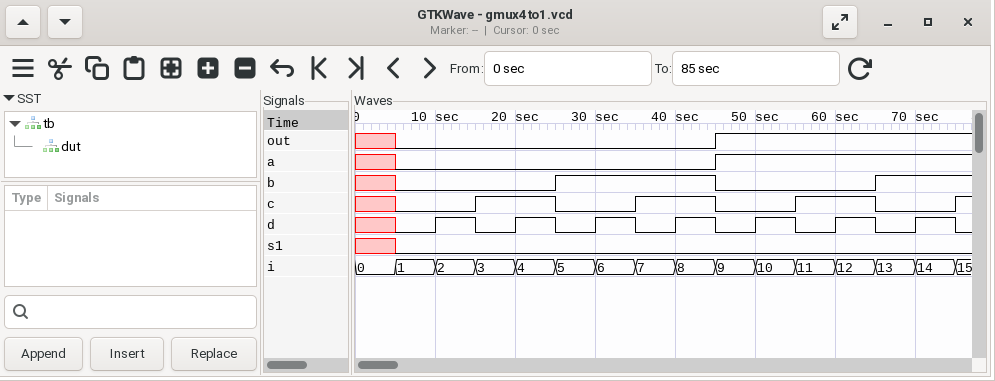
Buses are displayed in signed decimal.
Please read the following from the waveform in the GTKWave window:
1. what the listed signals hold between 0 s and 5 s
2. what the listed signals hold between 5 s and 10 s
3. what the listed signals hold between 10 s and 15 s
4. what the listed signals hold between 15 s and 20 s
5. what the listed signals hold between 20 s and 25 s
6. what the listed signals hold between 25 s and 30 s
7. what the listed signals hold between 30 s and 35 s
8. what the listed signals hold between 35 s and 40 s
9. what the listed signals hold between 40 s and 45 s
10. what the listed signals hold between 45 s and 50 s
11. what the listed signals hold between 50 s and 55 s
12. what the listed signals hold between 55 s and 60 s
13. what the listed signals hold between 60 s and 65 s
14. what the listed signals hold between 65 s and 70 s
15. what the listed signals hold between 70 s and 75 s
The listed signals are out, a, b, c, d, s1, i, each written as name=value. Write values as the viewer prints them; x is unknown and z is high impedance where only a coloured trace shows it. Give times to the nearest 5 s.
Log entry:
out=x, a=x, b=x, c=x, d=x, s1=x, i=0
out=0, a=0, b=0, c=0, d=0, s1=0, i=1
out=0, a=0, b=0, c=0, d=1, s1=0, i=2
out=0, a=0, b=0, c=1, d=0, s1=0, i=3
out=0, a=0, b=0, c=1, d=1, s1=0, i=4
out=0, a=0, b=1, c=0, d=0, s1=0, i=5
out=0, a=0, b=1, c=0, d=1, s1=0, i=6
out=0, a=0, b=1, c=1, d=0, s1=0, i=7
out=0, a=0, b=1, c=1, d=1, s1=0, i=8
out=1, a=1, b=0, c=0, d=0, s1=0, i=9
out=1, a=1, b=0, c=0, d=1, s1=0, i=10
out=1, a=1, b=0, c=1, d=0, s1=0, i=11
out=1, a=1, b=0, c=1, d=1, s1=0, i=12
out=1, a=1, b=1, c=0, d=0, s1=0, i=13
out=1, a=1, b=1, c=0, d=1, s1=0, i=14
